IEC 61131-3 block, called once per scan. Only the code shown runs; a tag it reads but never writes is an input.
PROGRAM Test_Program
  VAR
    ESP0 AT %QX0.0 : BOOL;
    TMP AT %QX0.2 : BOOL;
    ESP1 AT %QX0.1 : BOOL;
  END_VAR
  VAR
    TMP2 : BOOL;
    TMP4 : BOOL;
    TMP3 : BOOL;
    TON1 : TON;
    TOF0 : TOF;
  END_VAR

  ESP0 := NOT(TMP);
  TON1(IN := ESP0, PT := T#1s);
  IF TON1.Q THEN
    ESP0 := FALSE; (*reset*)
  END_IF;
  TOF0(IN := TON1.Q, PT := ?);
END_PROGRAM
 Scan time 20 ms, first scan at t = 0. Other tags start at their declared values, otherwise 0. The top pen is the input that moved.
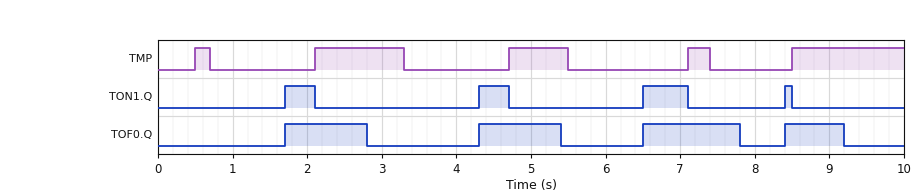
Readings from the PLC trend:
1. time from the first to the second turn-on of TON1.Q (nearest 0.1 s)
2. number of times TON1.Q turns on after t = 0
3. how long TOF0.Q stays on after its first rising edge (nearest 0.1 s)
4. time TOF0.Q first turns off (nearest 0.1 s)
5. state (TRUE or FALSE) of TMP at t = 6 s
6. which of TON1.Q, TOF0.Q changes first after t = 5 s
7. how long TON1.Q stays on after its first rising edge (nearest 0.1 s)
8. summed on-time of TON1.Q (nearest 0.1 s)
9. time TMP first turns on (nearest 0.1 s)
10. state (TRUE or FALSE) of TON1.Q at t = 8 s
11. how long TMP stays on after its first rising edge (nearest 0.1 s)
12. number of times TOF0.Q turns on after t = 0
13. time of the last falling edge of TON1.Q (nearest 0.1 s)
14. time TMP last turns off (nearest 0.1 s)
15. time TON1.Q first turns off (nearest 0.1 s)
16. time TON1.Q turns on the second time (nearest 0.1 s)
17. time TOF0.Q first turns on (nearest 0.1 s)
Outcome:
2.6 s
4
1.1 s
2.8 s
FALSE
TOF0.Q
0.4 s
1.5 s
0.5 s
FALSE
0.2 s
4
8.5 s
7.4 s
2.1 s
4.3 s
1.7 s
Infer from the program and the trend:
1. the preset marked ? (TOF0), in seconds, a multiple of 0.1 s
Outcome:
0.7 s
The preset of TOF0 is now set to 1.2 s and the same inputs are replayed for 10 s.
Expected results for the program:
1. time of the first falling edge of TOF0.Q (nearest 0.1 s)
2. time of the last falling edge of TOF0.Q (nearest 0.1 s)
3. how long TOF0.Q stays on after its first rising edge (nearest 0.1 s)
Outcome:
3.3 s
9.7 s
1.6 s
